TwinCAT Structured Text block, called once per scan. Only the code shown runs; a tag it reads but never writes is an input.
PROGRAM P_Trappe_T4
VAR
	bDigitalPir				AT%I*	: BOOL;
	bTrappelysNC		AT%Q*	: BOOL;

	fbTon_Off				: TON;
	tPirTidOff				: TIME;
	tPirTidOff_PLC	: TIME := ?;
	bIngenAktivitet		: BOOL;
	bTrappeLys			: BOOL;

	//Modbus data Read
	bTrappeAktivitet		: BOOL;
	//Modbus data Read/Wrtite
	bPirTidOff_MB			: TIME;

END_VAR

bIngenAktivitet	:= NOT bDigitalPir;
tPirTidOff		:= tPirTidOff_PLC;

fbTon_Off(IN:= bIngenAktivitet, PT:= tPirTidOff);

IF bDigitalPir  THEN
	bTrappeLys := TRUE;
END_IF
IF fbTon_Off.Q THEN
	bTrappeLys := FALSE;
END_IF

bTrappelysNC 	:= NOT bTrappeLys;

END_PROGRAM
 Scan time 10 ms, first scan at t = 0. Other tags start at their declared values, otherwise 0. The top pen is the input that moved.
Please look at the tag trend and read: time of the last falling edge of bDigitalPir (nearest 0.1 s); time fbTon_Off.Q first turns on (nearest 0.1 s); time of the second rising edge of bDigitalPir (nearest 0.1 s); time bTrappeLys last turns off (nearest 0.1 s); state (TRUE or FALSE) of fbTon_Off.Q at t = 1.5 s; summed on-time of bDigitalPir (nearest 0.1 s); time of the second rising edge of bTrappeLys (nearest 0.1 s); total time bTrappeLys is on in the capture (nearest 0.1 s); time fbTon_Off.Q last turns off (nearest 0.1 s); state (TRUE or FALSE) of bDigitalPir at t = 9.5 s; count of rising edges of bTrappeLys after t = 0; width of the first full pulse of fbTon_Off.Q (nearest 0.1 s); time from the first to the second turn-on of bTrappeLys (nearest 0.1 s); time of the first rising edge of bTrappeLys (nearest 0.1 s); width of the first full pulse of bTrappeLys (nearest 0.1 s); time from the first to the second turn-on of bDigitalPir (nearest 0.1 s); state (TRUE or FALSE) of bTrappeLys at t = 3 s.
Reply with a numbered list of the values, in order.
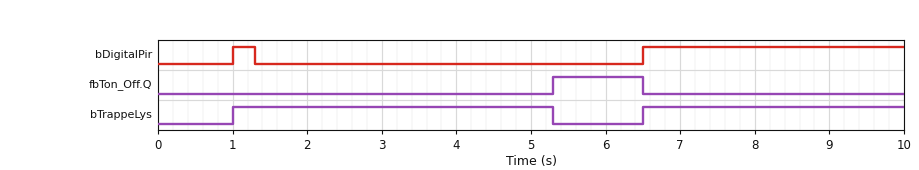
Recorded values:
1. 1.3 s
2. 5.3 s
3. 6.5 s
4. 5.3 s
5. FALSE
6. 3.8 s
7. 6.5 s
8. 7.8 s
9. 6.5 s
10. TRUE
11. 2
12. 1.2 s
13. 5.5 s
14. 1.0 s
15. 4.3 s
16. 5.5 s
17. TRUE
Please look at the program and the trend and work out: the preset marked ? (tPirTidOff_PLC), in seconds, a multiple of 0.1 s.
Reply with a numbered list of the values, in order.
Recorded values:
1. 4.0 s
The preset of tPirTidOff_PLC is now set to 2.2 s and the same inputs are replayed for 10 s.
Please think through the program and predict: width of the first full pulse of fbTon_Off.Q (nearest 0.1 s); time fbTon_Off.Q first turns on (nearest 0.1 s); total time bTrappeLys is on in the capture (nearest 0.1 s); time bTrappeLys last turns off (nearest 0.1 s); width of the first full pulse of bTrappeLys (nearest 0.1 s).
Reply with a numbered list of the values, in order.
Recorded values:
1. 3.0 s
2. 3.5 s
3. 6.0 s
4. 3.5 s
5. 2.5 s
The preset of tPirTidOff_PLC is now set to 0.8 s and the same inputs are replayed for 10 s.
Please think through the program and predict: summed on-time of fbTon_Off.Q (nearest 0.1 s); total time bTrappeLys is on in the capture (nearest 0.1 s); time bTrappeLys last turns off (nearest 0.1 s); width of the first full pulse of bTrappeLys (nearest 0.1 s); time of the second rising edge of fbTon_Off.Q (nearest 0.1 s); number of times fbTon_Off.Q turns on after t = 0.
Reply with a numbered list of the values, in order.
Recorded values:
1. 4.6 s
2. 4.6 s
3. 2.1 s
4. 1.1 s
5. 2.1 s
6. 2
